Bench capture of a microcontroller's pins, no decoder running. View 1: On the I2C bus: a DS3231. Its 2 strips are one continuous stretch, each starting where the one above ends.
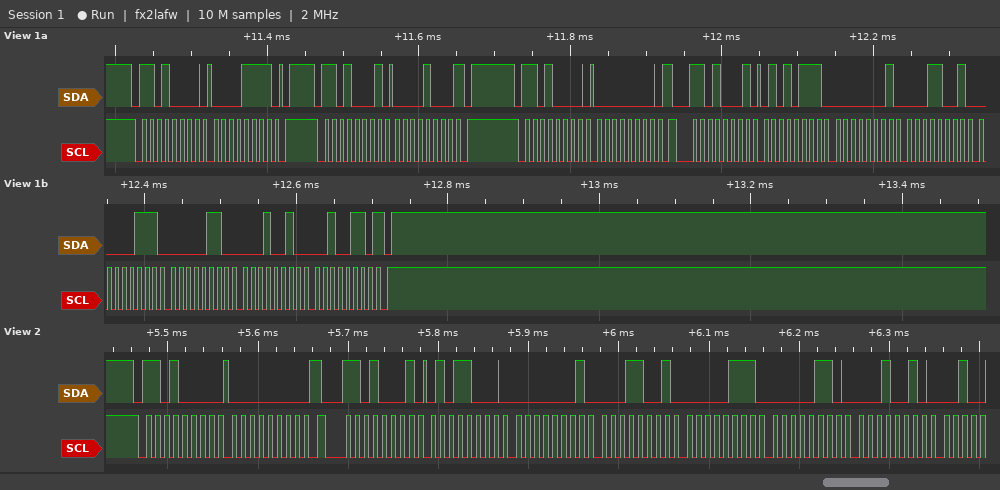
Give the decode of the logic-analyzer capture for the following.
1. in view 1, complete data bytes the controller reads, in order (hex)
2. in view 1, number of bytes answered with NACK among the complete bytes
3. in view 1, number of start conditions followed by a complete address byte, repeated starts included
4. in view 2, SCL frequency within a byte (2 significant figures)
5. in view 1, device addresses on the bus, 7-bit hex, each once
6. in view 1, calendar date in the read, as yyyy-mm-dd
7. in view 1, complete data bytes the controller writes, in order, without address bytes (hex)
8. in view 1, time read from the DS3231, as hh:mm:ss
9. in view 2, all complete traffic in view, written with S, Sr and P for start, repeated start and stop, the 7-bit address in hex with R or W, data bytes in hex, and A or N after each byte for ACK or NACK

08 57 01 19 07 06 12 26
2
4
100 kHz
0x68
2026-12-06
0F 00
19:01:57
S 68W A 00 A Sr 68R A 58 A 01 A 19 A 07 A 06 A 12 A
